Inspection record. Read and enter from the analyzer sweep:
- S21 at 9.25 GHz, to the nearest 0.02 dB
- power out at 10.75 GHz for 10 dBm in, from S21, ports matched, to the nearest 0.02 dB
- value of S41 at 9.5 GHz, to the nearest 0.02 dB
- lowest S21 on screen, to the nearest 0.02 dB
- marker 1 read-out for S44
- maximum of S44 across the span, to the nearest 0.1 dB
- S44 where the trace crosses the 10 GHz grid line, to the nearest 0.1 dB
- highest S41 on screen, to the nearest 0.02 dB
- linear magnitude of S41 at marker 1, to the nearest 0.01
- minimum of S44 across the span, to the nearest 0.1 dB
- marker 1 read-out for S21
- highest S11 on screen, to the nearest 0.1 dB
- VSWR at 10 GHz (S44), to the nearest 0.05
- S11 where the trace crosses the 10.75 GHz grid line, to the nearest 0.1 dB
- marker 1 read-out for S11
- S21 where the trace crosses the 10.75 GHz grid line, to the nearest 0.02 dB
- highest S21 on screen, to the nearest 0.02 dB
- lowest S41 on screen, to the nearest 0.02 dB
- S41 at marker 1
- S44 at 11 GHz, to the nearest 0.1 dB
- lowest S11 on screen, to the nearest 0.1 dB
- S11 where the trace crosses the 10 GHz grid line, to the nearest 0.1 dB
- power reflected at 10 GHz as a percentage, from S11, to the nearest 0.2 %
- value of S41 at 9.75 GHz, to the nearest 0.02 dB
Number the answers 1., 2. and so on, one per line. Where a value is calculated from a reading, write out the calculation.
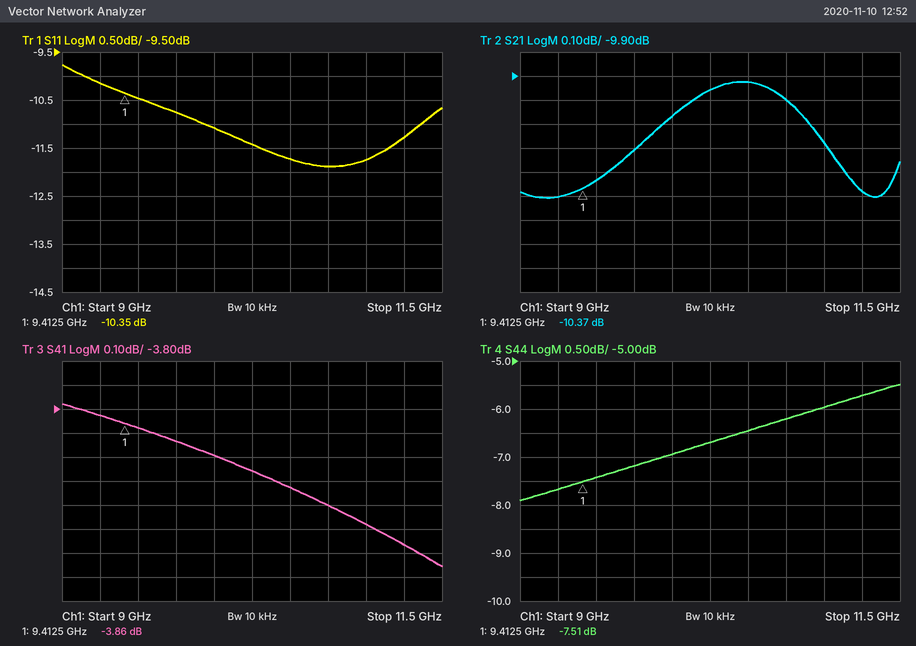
1. -10.40 dB
2. 10 dBm + (-10.00 dB) = 0.00 dBm
3. -3.88 dB
4. -10.40 dB
5. -7.51 dB
6. -5.5 dB
7. -6.9 dB
8. -3.78 dB
9. 10^(-3.86/20) ≈ 0.64
10. -7.9 dB
11. -10.37 dB
12. -9.8 dB
13. |Γ| = 10^(-6.9/20) = 0.4519; VSWR = (1 + 0.4519)/(1 − 0.4519) ≈ 2.65
14. -11.9 dB
15. -10.35 dB
16. -10.00 dB
17. -9.92 dB
18. -4.46 dB
19. -3.86 dB
20. -6.0 dB
21. -11.9 dB
22. -11.1 dB
23. 10^(-11.1/10) ≈ 7.8 %
24. -3.94 dB
